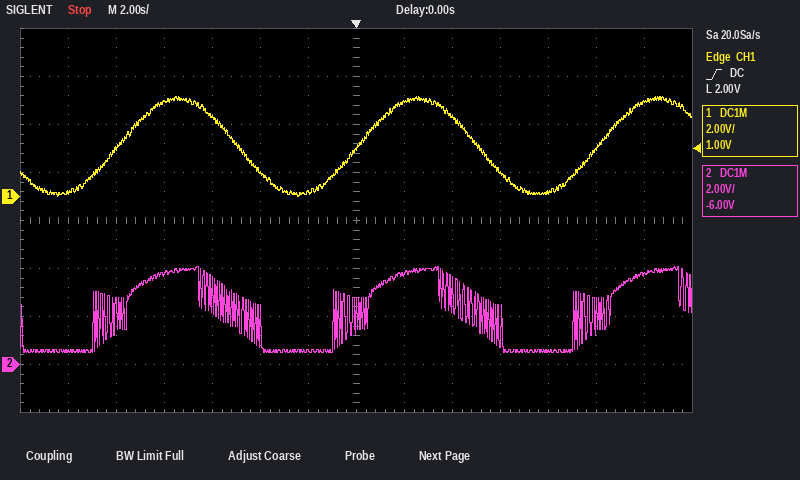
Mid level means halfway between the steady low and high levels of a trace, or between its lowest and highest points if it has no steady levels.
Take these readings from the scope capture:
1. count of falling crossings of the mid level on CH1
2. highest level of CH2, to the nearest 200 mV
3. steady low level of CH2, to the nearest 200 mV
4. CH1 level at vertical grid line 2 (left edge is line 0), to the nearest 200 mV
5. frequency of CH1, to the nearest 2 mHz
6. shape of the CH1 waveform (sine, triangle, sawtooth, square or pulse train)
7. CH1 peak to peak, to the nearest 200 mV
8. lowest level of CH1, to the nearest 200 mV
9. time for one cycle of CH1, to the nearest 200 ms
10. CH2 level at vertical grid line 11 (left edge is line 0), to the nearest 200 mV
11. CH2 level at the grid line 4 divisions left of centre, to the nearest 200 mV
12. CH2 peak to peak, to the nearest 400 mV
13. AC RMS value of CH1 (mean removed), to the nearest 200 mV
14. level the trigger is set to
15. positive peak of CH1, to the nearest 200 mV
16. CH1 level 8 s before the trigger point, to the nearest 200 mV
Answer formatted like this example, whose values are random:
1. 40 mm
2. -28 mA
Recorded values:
1. 2
2. 4.0 V
3. 600 mV
4. 2.0 V
5. 100 mHz
6. sine
7. 4.2 V
8. 0.0 V
9. 10.0 s
10. 600 mV
11. 3.8 V
12. 3.6 V
13. 1.4 V
14. 2.00 V
15. 4.2 V
16. 4.0 V
